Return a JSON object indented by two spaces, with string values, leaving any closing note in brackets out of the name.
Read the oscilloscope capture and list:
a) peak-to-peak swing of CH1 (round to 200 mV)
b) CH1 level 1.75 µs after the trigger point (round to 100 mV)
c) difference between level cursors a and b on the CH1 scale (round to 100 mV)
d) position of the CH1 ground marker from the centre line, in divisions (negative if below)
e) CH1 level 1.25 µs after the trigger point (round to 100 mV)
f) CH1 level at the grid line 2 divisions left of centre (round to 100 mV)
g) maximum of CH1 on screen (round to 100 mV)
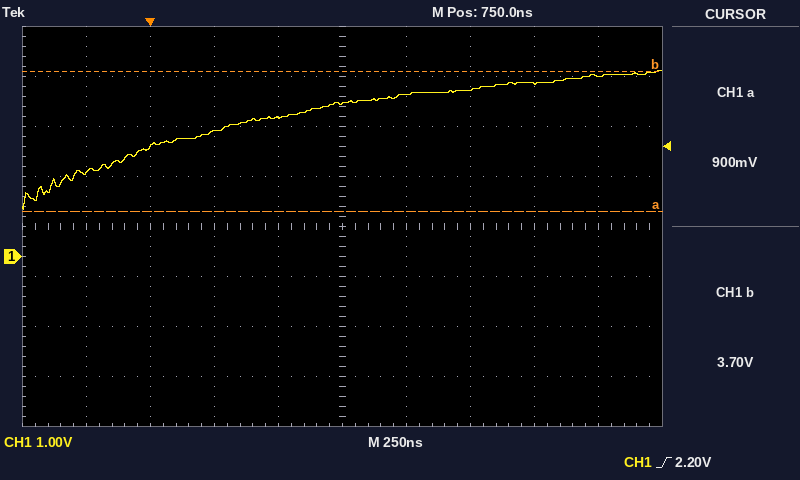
{
  "peak-to-peak swing of CH1": "2.8 V",
  "CH1 level 1.75 µs after the trigger point": "3.6 V",
  "difference between level cursors a and b on the CH1 scale": "2.8 V",
  "position of the CH1 ground marker from the centre line, in divisions": "-0.6 div",
  "CH1 level 1.25 µs after the trigger point": "3.3 V",
  "CH1 level at the grid line 2 divisions left of centre": "2.5 V",
  "maximum of CH1 on screen": "3.7 V"
}
